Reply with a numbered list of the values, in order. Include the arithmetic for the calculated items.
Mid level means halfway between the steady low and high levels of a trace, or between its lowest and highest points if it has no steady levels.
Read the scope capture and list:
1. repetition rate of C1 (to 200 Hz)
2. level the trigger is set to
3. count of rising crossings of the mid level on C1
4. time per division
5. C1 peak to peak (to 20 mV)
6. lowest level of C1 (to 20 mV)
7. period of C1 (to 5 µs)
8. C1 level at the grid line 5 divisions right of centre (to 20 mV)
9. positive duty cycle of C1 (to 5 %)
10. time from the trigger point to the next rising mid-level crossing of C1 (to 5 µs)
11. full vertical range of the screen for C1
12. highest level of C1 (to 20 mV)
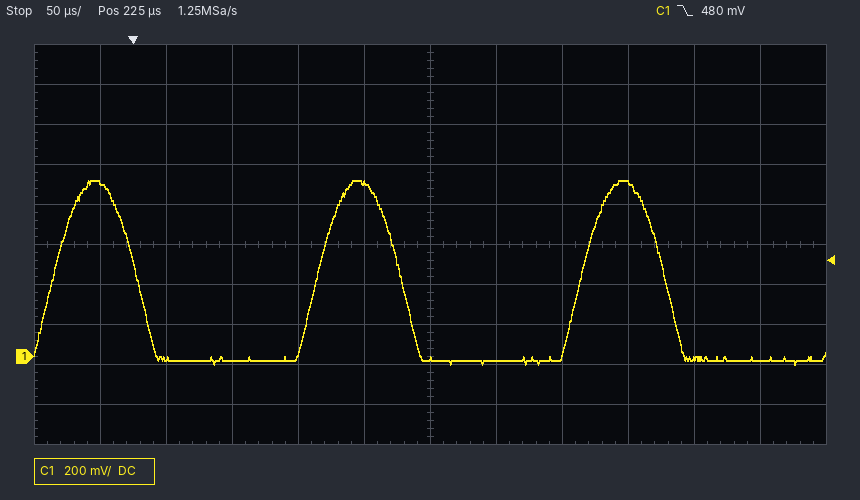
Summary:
1. 1 / 200 µs ≈ 5.0 kHz
2. 480 mV
3. 3
4. 50 µs
5. 880 mV − (-40 mV) = 920 mV
6. -40 mV
7. 200 µs
8. -20 mV
9. 30 %
10. 140 µs
11. 2 V
12. 880 mV
